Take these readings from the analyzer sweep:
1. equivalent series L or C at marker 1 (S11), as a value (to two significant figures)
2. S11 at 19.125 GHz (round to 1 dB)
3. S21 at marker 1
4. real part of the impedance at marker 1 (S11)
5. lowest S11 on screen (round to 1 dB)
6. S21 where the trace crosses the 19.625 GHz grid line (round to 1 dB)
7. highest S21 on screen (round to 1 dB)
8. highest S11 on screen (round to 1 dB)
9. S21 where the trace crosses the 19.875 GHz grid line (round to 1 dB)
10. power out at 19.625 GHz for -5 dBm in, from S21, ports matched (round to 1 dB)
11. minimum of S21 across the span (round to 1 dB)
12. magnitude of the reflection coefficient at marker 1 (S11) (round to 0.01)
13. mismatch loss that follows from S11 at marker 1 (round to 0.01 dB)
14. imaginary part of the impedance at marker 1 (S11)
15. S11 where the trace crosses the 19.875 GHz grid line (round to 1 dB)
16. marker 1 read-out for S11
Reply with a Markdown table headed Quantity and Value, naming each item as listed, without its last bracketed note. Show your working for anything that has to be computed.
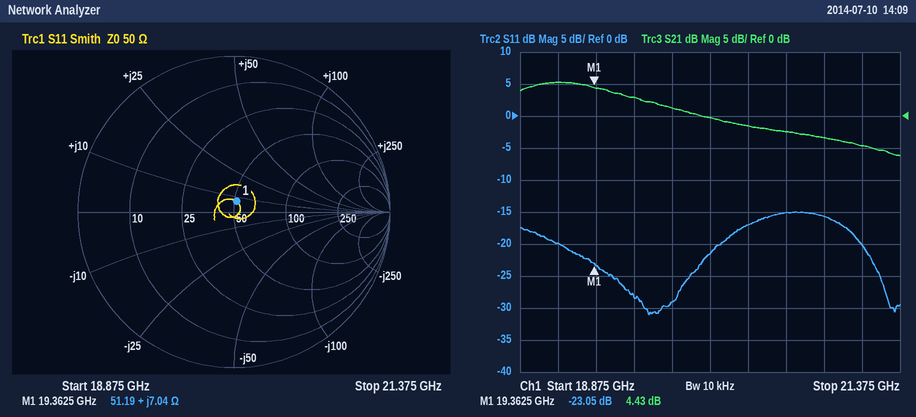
| Quantity | Value |
|---|---|
| equivalent series L or C at marker 1 (S11), as a value | L = 7.04 Ω/(2π × 19.3625 GHz) ≈ 58 pH |
| S11 at 19.125 GHz | -20 dB |
| S21 at marker 1 | 4.43 dB |
| real part of the impedance at marker 1 | 51.19 Ω |
| lowest S11 on screen | -31 dB |
| S21 where the trace crosses the 19.625 GHz grid line | 3 dB |
| highest S21 on screen | 5 dB |
| highest S11 on screen | -15 dB |
| S21 where the trace crosses the 19.875 GHz grid line | 1 dB |
| power out at 19.625 GHz for -5 dBm in, from S21, ports matched | -5 dBm + (3 dB) = -2 dBm |
| minimum of S21 across the span | -6 dB |
| magnitude of the reflection coefficient at marker 1 (S11) | 0.07 |
| mismatch loss that follows from S11 at marker 1 | −10 log10(1 − 10^(-23.05/10)) ≈ 0.02 dB |
| imaginary part of the impedance at marker 1 | +7.04 Ω |
| S11 where the trace crosses the 19.875 GHz grid line | -29 dB |
| marker 1 read-out for S11 | -23.05 dB |
